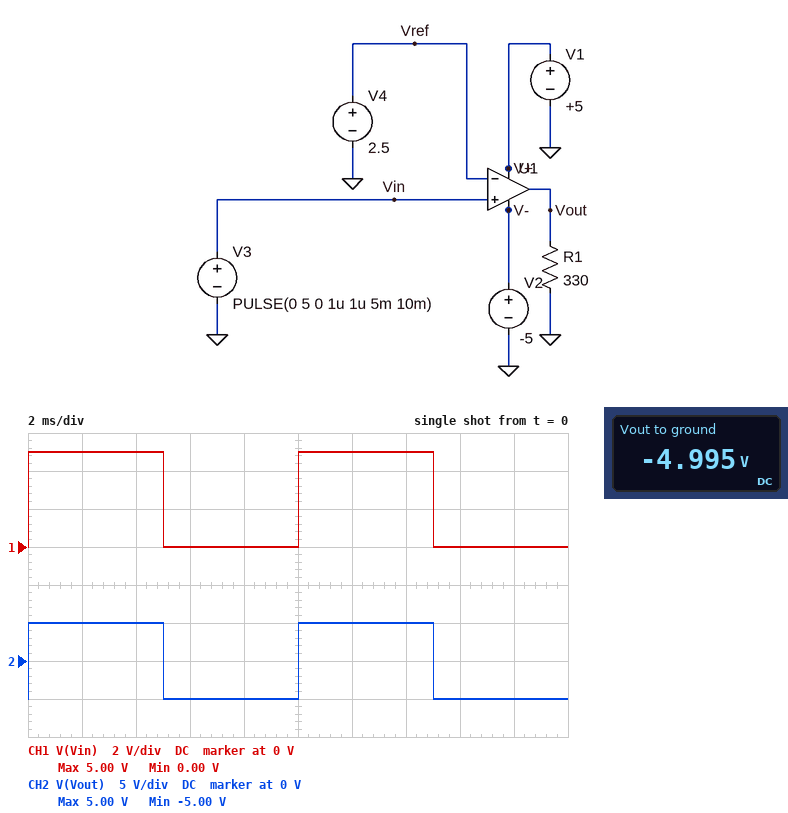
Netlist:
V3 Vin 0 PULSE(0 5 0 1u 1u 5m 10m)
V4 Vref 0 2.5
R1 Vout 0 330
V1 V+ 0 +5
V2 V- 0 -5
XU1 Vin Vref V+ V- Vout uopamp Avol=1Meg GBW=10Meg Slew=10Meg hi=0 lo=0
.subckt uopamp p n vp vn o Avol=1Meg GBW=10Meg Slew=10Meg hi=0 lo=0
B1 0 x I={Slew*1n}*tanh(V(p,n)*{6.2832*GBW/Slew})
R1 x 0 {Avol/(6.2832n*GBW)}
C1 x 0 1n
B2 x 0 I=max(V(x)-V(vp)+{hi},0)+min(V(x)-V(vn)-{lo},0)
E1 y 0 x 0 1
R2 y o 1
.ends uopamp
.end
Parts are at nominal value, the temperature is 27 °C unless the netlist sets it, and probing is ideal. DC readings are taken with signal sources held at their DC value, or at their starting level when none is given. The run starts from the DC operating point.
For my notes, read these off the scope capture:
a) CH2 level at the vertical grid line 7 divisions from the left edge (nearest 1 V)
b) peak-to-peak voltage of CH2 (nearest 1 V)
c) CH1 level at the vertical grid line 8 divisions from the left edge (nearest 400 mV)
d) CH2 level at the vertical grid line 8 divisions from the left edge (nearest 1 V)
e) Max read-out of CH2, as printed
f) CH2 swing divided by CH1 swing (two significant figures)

5 V
10 V
0 V
-5 V
5.00 V
2.0
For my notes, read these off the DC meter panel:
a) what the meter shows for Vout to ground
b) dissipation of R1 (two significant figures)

-4.995 V
76 mW
